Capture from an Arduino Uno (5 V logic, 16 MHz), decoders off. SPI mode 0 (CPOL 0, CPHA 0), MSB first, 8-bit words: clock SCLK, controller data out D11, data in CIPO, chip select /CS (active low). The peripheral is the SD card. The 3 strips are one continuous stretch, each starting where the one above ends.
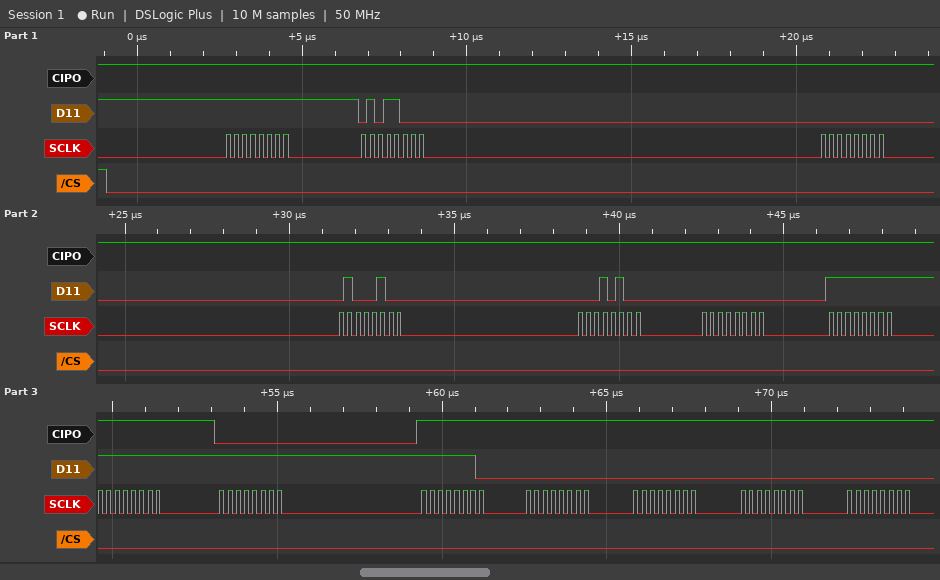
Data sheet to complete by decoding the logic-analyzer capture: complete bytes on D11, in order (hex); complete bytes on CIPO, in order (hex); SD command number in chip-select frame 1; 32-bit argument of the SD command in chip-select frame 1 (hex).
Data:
FF 58 00 44 14 00 FF FF FF FE 00 00 00 00
FF FF FF FF FF FF FF FF 00 FF FF FF FF FF
CMD24
0x00441400
